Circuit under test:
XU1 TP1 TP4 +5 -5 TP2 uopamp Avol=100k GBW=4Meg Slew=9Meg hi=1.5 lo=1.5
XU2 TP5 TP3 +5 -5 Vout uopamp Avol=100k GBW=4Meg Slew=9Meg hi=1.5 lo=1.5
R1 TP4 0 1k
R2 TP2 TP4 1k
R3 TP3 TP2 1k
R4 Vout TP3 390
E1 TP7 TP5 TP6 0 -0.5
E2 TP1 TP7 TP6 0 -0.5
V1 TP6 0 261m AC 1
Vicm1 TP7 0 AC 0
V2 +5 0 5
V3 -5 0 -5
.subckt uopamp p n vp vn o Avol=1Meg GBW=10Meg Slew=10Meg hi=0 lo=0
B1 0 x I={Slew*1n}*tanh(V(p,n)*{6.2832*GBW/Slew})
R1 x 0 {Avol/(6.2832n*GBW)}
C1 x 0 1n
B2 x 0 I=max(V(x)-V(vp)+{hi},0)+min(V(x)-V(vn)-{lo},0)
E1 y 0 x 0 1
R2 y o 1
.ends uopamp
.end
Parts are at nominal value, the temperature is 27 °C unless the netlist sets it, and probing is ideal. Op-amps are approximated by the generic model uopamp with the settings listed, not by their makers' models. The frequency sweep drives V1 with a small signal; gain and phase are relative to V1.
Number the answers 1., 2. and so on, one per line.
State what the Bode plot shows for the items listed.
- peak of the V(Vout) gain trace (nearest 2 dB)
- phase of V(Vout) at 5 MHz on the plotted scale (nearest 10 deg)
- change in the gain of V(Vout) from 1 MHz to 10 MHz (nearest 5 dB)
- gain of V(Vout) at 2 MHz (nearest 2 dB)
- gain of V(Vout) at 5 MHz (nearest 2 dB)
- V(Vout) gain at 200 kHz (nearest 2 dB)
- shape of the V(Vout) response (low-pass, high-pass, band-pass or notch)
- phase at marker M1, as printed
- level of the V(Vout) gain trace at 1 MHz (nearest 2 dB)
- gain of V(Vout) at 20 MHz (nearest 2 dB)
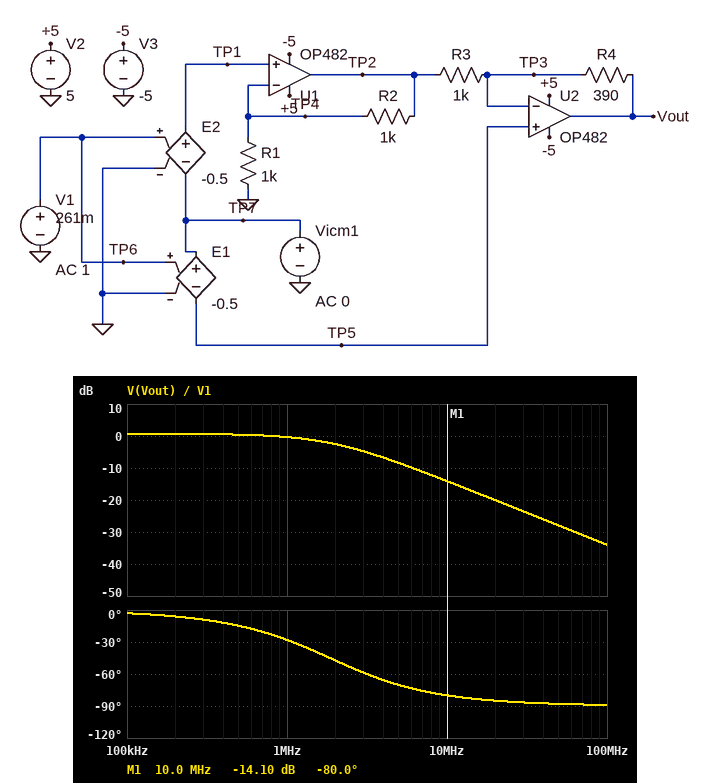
1. 0 dB
2. -70 deg
3. -15 dB
4. -2 dB
5. -8 dB
6. 0 dB
7. low-pass
8. -80.0 deg
9. 0 dB
10. -20 dB
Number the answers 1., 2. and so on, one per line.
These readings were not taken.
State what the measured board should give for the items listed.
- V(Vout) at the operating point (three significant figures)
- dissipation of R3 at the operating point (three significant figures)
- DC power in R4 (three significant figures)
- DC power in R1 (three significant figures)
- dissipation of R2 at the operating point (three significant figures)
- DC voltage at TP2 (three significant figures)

1. 283 mV
2. 153 µW
3. 59.8 µW
4. 17.0 µW
5. 17.0 µW
6. -261 mV
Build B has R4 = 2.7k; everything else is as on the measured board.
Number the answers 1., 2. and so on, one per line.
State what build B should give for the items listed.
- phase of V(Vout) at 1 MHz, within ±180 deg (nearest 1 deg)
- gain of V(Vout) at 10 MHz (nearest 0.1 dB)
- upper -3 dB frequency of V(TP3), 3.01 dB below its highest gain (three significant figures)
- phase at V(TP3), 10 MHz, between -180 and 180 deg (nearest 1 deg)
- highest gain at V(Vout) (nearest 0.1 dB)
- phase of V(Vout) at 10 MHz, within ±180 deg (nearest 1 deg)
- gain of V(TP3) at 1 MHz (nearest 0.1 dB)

1. -58 deg
2. -13.3 dB
3. 1.76 MHz
4. 114 deg
5. 13.2 dB
6. -99 deg
7. -7.3 dB
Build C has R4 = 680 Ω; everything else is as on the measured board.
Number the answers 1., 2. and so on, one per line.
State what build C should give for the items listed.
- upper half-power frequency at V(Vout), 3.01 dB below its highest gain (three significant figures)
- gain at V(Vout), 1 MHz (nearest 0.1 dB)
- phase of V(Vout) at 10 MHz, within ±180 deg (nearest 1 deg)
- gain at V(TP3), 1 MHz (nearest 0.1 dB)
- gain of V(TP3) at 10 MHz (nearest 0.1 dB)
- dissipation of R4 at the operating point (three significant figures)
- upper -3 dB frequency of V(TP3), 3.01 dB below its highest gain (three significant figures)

1. 1.60 MHz
2. 2.3 dB
3. -85 deg
4. -7.6 dB
5. -27.4 dB
6. 104 µW
7. 1.46 MHz
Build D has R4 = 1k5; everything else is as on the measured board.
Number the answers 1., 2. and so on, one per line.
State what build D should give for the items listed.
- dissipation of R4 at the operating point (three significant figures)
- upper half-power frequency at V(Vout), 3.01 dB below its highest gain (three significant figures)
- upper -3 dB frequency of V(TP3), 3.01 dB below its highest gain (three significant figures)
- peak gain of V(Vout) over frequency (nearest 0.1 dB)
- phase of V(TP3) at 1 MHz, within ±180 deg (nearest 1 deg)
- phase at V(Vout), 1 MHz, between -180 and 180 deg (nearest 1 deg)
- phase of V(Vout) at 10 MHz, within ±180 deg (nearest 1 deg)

1. 230 µW
2. 1.21 MHz
3. 1.23 MHz
4. 8.8 dB
5. -73 deg
6. -46 deg
7. -93 deg
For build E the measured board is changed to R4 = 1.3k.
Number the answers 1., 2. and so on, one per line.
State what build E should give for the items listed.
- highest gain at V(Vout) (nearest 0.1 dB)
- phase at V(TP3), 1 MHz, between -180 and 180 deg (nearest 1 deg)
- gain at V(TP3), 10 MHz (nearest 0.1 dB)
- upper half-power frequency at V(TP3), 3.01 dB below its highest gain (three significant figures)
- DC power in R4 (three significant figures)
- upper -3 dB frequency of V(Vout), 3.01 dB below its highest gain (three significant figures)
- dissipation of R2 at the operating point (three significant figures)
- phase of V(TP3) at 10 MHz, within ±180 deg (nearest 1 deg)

1. 7.8 dB
2. -65 deg
3. -30.4 dB
4. 1.23 MHz
5. 199 µW
6. 1.28 MHz
7. 17.0 µW
8. 145 deg
